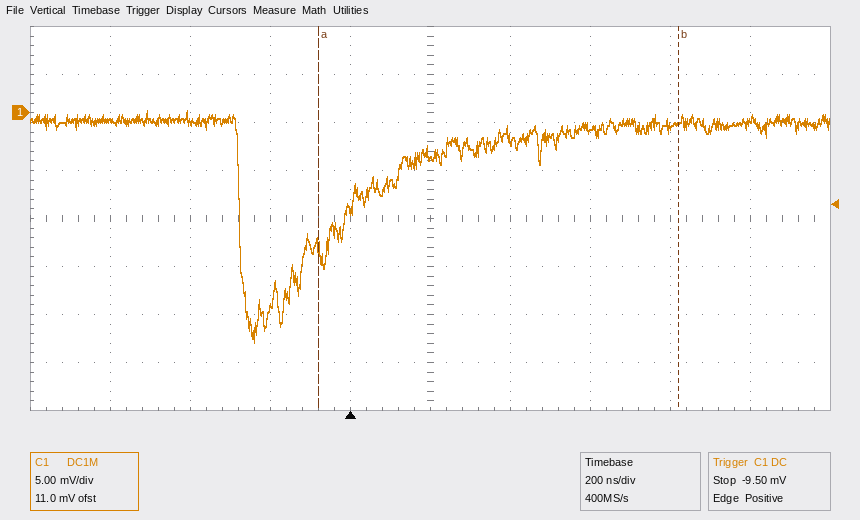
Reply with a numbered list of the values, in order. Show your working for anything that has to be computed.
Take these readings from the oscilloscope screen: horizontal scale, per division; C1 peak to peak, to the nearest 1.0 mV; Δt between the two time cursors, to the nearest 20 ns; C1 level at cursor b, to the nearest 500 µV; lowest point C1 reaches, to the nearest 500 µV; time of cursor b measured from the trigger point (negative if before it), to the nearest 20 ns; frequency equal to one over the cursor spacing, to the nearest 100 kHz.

1. 200 ns
2. 24.0 mV
3. 900 ns
4. -1.0 mV
5. -24.0 mV
6. +820 ns
7. 1 / 900 ns ≈ 1.1 MHz
